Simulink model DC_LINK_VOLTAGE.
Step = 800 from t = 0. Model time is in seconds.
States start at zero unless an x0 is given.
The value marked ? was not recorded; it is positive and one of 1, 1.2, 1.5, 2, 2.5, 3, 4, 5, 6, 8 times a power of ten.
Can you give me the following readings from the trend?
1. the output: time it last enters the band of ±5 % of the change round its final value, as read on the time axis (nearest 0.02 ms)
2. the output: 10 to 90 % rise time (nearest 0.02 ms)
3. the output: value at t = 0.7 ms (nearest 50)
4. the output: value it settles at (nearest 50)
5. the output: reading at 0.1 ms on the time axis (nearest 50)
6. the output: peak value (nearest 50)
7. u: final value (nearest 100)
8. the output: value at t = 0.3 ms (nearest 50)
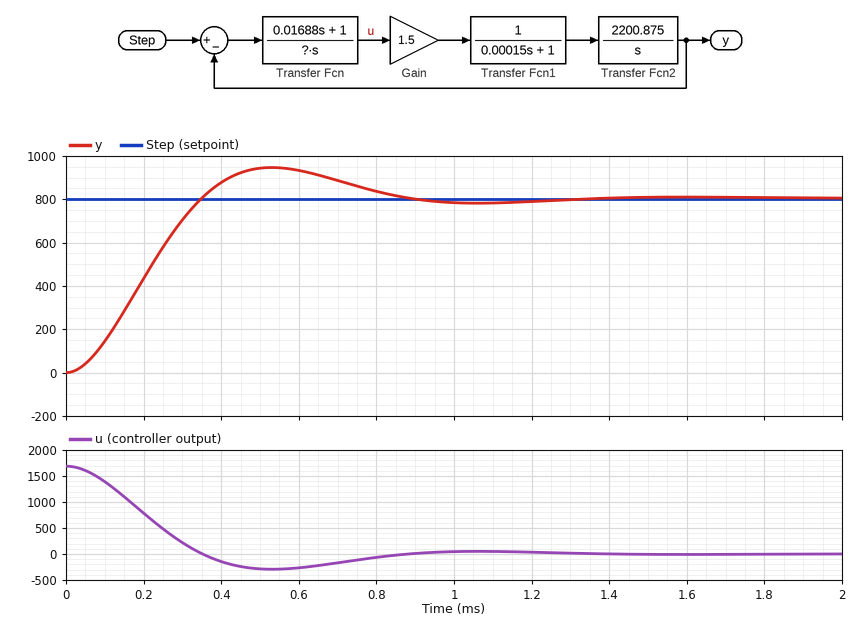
0.78 ms
0.24 ms
900
800
150
950
0
700
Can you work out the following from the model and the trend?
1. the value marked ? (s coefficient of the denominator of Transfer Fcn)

0.008
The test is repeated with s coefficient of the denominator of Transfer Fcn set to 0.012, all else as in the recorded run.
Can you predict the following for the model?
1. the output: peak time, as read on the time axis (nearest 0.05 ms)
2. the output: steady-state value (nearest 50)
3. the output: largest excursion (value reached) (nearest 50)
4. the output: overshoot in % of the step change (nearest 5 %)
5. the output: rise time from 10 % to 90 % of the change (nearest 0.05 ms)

0.70 ms
800
900
10 %
0.35 ms
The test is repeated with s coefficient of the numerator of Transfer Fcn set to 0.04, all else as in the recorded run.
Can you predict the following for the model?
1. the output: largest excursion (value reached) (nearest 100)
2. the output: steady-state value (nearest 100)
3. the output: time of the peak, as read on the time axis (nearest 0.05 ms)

1100
800
0.30 ms
